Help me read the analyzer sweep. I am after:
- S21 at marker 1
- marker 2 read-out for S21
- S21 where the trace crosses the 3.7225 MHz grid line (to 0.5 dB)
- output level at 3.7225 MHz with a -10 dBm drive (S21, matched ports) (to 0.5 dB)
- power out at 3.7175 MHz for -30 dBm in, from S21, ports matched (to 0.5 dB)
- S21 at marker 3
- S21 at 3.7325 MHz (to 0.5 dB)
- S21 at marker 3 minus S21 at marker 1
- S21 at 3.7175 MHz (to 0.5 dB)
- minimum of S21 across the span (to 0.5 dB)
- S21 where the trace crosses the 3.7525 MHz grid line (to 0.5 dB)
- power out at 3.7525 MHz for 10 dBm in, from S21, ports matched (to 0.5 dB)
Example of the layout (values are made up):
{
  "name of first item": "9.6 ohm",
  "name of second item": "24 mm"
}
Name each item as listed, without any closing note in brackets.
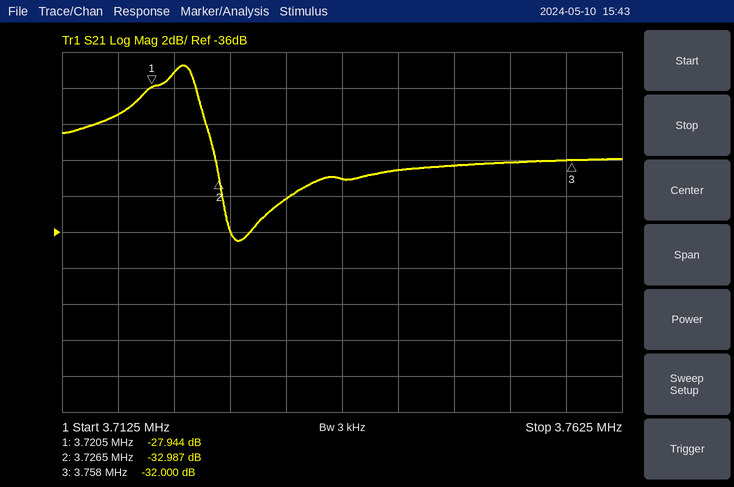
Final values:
{
  "S21 at marker 1": "-27.944 dB",
  "marker 2 read-out for S21": "-32.987 dB",
  "S21 where the trace crosses the 3.7225 MHz grid line": "-27.0 dB",
  "output level at 3.7225 MHz with a -10 dBm drive (S21, matched ports)": "-37.0 dBm",
  "power out at 3.7175 MHz for -30 dBm in, from S21, ports matched": "-59.5 dBm",
  "S21 at marker 3": "-32.000 dB",
  "S21 at 3.7325 MHz": "-34.0 dB",
  "S21 at marker 3 minus S21 at marker 1": "-4.056 dB",
  "S21 at 3.7175 MHz": "-29.5 dB",
  "minimum of S21 across the span": "-36.5 dB",
  "S21 where the trace crosses the 3.7525 MHz grid line": "-32.0 dB",
  "power out at 3.7525 MHz for 10 dBm in, from S21, ports matched": "-22.0 dBm"
}
